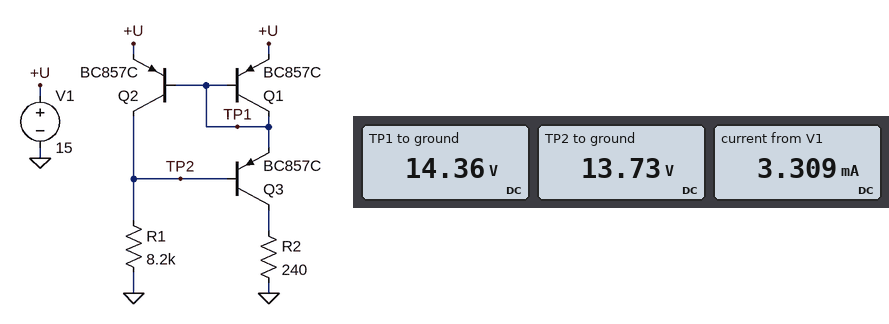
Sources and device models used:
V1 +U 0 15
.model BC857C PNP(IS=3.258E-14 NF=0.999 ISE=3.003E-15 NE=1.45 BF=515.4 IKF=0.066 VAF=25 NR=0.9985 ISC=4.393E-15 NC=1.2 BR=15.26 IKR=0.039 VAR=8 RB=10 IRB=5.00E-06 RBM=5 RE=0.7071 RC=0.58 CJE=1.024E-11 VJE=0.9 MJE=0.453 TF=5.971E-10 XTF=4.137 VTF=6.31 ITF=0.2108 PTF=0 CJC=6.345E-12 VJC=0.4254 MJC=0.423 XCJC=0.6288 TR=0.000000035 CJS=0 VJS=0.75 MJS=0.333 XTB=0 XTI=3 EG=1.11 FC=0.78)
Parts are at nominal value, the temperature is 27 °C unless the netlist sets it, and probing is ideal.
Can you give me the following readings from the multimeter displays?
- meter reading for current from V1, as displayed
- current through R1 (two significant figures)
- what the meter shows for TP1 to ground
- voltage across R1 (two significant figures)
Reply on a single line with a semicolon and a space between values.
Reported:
3.309 mA; 1.7 mA; 14.36 V; 14 V
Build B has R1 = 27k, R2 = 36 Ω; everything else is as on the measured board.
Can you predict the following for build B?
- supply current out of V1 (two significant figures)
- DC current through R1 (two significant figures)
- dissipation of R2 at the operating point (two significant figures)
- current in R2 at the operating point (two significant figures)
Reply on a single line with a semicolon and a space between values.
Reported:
1.0 mA; 510 µA; 9.0 µW; 500 µA
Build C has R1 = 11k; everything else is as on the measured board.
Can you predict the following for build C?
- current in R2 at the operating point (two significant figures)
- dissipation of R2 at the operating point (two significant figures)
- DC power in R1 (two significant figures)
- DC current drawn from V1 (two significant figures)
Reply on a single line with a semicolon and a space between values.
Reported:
1.2 mA; 360 µW; 17 mW; 2.5 mA
